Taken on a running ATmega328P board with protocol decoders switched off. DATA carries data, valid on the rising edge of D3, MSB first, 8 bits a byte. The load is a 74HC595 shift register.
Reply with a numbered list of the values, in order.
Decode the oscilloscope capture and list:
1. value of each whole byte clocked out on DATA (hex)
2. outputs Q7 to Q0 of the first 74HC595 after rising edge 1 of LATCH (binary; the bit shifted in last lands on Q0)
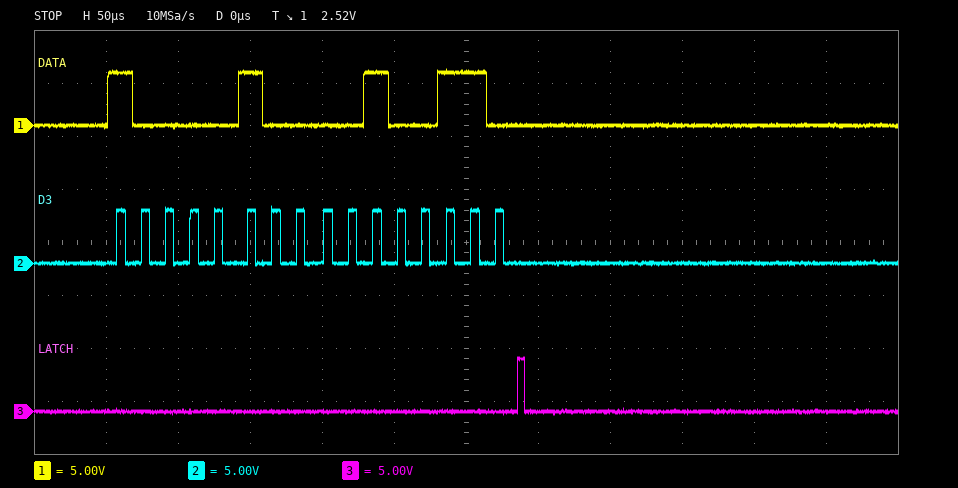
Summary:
1. 0x84 0x26
2. 00100110
